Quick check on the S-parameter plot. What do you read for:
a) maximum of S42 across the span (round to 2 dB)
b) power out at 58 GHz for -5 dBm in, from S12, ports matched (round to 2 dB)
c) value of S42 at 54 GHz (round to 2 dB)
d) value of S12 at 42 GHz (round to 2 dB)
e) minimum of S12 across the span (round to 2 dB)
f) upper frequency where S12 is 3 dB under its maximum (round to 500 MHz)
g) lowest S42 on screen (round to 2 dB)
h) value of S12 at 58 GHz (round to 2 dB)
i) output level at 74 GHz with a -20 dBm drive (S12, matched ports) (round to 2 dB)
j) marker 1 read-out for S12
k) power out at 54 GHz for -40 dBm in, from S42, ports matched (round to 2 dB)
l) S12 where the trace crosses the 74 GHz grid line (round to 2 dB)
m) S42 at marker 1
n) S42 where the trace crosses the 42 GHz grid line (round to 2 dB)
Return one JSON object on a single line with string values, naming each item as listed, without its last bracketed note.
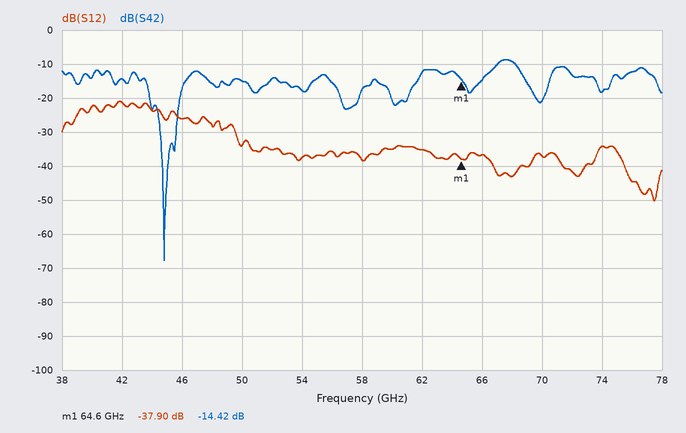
{"maximum of S42 across the span": "-8 dB", "power out at 58 GHz for -5 dBm in, from S12, ports matched": "-44 dBm", "value of S42 at 54 GHz": "-18 dB", "value of S12 at 42 GHz": "-22 dB", "minimum of S12 across the span": "-50 dB", "upper frequency where S12 is 3 dB under its maximum": "44.5 GHz", "lowest S42 on screen": "-68 dB", "value of S12 at 58 GHz": "-38 dB", "output level at 74 GHz with a -20 dBm drive (S12, matched ports)": "-54 dBm", "marker 1 read-out for S12": "-37.90 dB", "power out at 54 GHz for -40 dBm in, from S42, ports matched": "-58 dBm", "S12 where the trace crosses the 74 GHz grid line": "-34 dB", "S42 at marker 1": "-14.42 dB", "S42 where the trace crosses the 42 GHz grid line": "-14 dB"}
